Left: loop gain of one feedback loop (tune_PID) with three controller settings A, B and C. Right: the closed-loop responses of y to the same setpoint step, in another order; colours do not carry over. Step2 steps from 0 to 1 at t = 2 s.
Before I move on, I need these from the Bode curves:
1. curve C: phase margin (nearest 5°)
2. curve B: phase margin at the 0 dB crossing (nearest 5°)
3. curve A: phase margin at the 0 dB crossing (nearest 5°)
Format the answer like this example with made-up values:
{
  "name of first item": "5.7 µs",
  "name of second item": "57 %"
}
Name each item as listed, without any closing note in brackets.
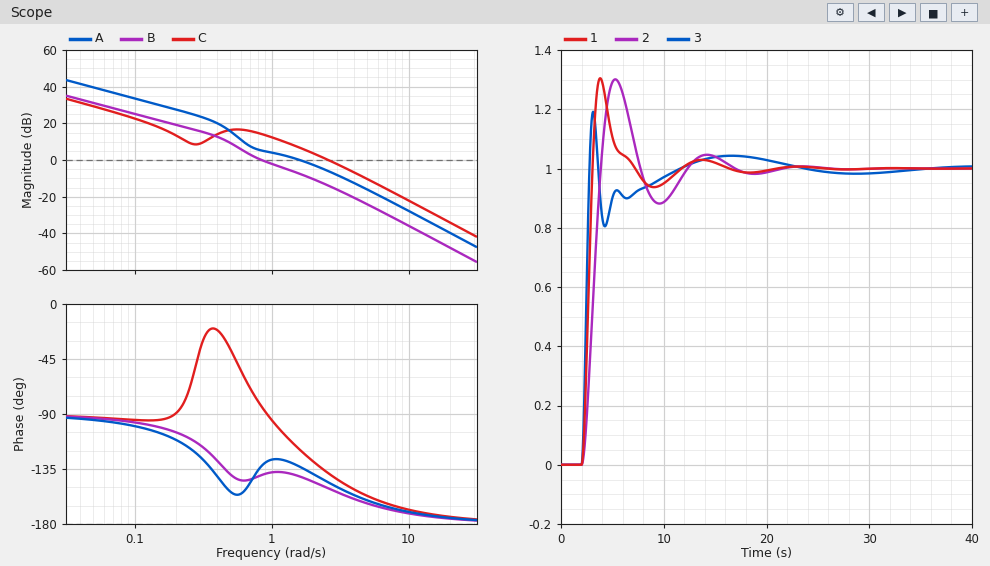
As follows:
{
  "curve C: phase margin": "40°",
  "curve B: phase margin at the 0 dB crossing": "40°",
  "curve A: phase margin at the 0 dB crossing": "45°"
}
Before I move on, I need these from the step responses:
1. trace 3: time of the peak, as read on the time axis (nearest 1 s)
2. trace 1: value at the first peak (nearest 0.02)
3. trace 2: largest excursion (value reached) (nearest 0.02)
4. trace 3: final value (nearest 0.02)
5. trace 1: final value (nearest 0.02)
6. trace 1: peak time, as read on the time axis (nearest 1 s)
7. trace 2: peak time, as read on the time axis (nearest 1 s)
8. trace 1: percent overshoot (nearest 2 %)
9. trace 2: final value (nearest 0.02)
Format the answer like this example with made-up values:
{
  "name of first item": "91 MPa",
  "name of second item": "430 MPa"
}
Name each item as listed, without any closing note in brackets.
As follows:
{
  "trace 3: time of the peak, as read on the time axis": "3 s",
  "trace 1: value at the first peak": "1.30",
  "trace 2: largest excursion (value reached)": "1.30",
  "trace 3: final value": "1.00",
  "trace 1: final value": "1.00",
  "trace 1: peak time, as read on the time axis": "4 s",
  "trace 2: peak time, as read on the time axis": "5 s",
  "trace 1: percent overshoot": "30 %",
  "trace 2: final value": "1.00"
}
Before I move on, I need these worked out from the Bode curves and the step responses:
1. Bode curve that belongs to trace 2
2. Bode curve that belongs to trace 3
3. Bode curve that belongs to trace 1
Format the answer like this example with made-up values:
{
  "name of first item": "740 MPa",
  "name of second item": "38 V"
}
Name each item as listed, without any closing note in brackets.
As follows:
{
  "Bode curve that belongs to trace 2": "B",
  "Bode curve that belongs to trace 3": "C",
  "Bode curve that belongs to trace 1": "A"
}
